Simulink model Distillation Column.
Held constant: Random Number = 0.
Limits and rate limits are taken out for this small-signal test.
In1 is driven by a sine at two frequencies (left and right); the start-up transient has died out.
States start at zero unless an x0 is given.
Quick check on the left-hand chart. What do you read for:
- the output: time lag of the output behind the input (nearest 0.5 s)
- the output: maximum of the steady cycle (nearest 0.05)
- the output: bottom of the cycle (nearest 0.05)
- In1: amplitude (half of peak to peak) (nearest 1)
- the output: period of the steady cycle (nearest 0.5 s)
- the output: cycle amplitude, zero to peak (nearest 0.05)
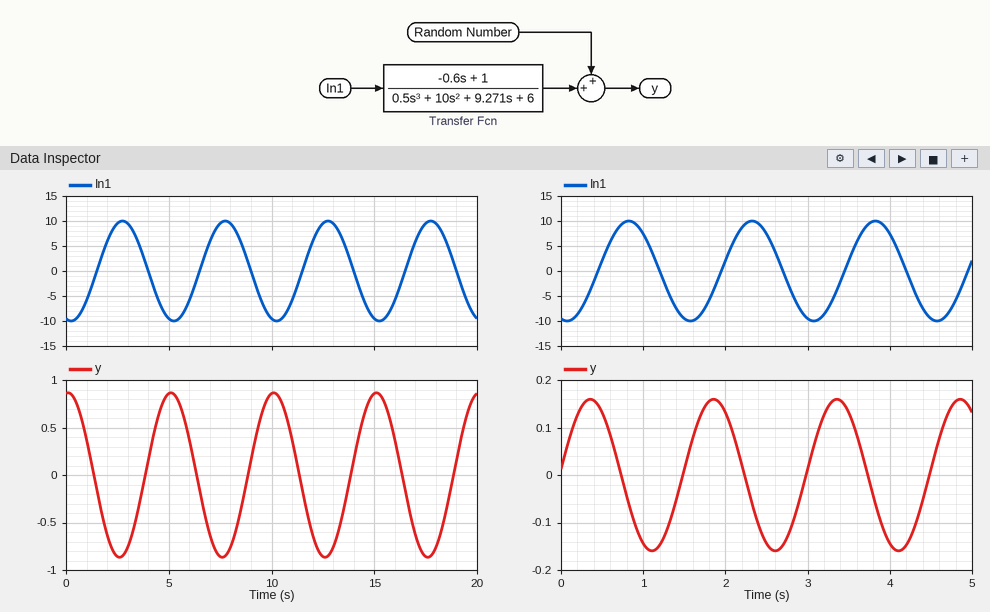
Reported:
2.5 s
0.85
-0.85
10
5.0 s
0.85
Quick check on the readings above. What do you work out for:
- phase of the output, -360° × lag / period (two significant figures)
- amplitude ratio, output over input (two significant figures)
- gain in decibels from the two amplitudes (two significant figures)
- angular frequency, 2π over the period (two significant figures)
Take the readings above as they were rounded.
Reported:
-180°
0.085
-21 dB
1.3 rad/s
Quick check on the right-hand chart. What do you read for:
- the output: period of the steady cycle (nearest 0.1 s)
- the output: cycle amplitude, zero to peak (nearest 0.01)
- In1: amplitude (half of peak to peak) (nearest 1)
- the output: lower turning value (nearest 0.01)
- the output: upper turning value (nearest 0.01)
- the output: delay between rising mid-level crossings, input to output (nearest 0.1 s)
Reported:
1.5 s
0.16
10
-0.16
0.16
1.0 s
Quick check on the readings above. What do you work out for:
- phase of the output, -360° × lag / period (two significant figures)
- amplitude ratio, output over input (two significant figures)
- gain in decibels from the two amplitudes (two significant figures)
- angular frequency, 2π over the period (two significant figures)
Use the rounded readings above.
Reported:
-240°
0.016
-36 dB
4.2 rad/s
